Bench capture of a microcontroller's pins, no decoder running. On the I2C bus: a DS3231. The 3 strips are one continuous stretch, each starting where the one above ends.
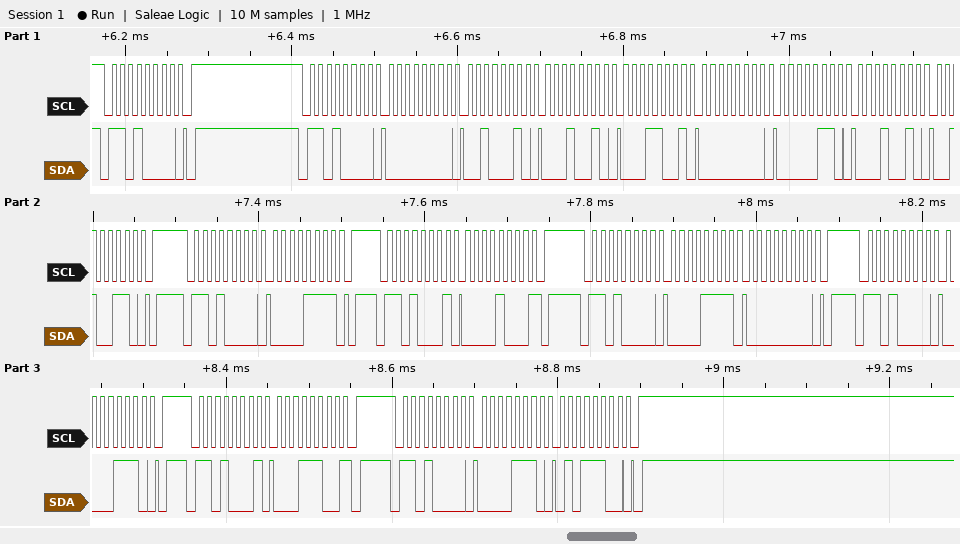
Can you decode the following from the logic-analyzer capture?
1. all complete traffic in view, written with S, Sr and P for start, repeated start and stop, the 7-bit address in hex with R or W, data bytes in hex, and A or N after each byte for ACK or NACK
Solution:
S 68W A P S 68W A 00 A 22 A 12 A 19 A 00 A 06 A 12 A 26 A P S 68W A 0F A P S 68R A 08 N P S 68W A 0F A 00 A P S 68W A 0E A P S 68R A 1C N P S 68W A 0E A 5C A P
